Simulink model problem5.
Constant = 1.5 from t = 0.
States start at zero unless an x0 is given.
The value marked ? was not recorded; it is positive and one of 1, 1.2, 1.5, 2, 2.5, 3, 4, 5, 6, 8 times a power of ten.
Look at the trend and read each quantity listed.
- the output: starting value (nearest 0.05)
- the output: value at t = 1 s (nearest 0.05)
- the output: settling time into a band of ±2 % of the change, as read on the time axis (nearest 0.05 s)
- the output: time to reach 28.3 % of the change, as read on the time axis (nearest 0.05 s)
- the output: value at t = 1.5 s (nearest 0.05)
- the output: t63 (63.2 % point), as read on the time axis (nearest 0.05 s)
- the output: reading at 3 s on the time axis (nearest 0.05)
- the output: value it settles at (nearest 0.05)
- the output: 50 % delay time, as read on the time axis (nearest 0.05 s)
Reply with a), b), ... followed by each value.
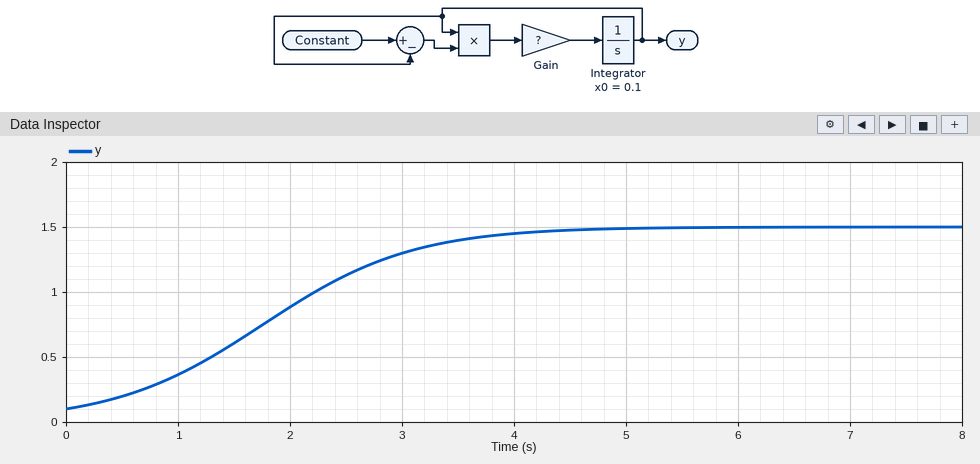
a) 0.10
b) 0.35
c) 4.40 s
d) 1.30 s
e) 0.60
f) 2.20 s
g) 1.30
h) 1.50
i) 1.85 s
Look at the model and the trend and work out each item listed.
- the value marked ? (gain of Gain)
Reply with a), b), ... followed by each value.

a) 1
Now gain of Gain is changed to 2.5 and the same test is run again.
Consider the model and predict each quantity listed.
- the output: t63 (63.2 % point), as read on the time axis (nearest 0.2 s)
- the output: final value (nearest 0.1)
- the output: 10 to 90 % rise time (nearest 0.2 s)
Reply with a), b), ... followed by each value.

a) 0.8 s
b) 1.5
c) 1.0 s
